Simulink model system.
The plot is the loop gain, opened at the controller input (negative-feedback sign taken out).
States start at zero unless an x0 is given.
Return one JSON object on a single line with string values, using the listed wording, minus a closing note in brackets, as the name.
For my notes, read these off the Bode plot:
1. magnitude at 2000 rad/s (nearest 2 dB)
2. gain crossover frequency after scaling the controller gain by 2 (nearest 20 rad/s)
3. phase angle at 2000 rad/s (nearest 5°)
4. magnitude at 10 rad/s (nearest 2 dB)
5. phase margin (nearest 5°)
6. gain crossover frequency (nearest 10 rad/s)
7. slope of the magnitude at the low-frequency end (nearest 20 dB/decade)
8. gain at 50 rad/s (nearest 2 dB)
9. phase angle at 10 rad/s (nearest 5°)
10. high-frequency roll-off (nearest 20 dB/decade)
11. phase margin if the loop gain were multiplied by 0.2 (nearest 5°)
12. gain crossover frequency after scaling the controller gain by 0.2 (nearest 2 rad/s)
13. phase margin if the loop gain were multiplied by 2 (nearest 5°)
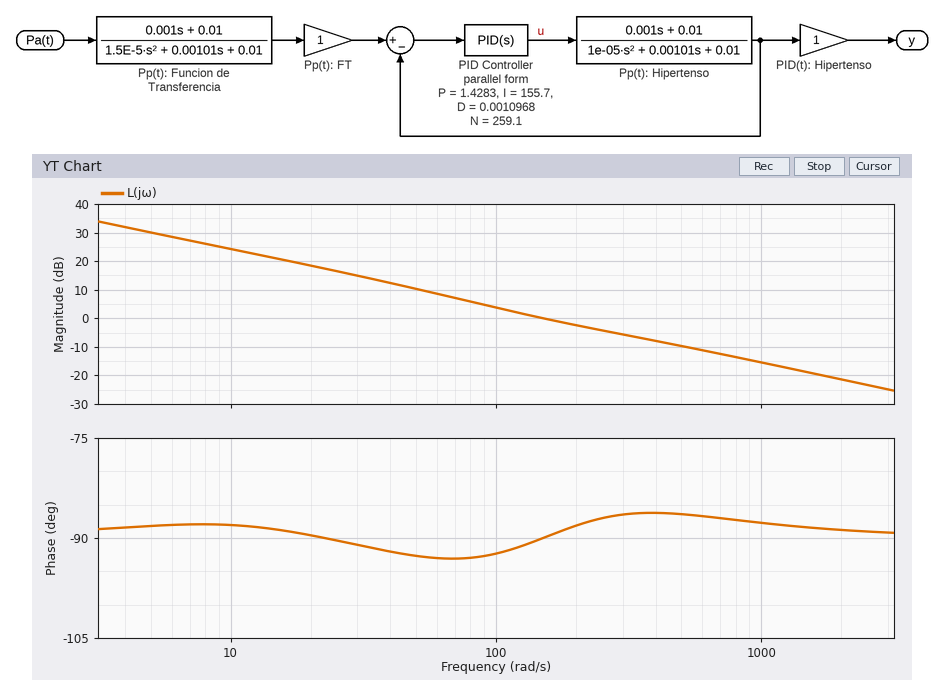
{"magnitude at 2000 rad/s": "-22 dB", "gain crossover frequency after scaling the controller gain by 2": "320 rad/s", "phase angle at 2000 rad/s": "-90°", "magnitude at 10 rad/s": "24 dB", "phase margin": "90°", "gain crossover frequency": "150 rad/s", "slope of the magnitude at the low-frequency end": "-20 dB/decade", "gain at 50 rad/s": "10 dB", "phase angle at 10 rad/s": "-90°", "high-frequency roll-off": "-20 dB/decade", "phase margin if the loop gain were multiplied by 0.2": "90°", "gain crossover frequency after scaling the controller gain by 0.2": "34 rad/s", "phase margin if the loop gain were multiplied by 2": "95°"}
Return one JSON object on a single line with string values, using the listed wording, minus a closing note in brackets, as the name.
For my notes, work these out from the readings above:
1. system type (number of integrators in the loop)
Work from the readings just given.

{"system type": "1"}
